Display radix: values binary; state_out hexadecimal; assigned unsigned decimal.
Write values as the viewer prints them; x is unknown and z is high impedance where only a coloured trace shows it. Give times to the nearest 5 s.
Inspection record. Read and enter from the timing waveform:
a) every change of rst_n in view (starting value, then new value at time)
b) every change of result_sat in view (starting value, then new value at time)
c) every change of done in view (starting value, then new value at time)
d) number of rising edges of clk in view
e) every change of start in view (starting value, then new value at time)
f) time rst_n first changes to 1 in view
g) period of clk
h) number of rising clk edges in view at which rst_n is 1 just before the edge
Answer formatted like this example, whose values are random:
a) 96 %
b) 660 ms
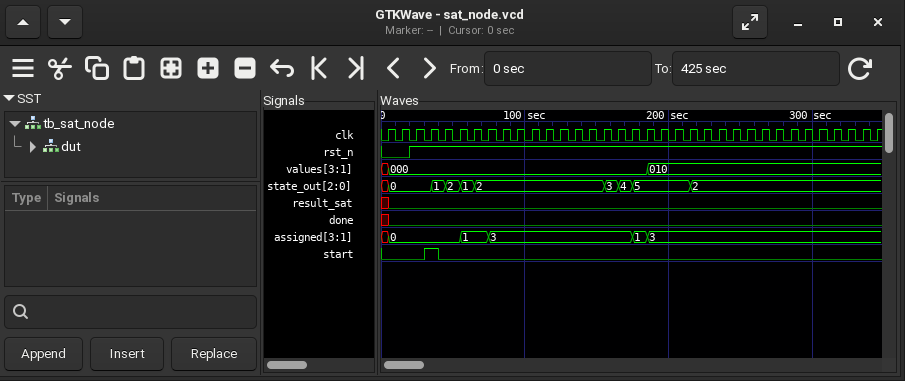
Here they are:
a) 0, 1 at 20 s
b) x, 0 at 5 s
c) x, 0 at 5 s
d) 35
e) 0, 1 at 30 s, 0 at 40 s
f) 20 s
g) 10 s
h) 33
